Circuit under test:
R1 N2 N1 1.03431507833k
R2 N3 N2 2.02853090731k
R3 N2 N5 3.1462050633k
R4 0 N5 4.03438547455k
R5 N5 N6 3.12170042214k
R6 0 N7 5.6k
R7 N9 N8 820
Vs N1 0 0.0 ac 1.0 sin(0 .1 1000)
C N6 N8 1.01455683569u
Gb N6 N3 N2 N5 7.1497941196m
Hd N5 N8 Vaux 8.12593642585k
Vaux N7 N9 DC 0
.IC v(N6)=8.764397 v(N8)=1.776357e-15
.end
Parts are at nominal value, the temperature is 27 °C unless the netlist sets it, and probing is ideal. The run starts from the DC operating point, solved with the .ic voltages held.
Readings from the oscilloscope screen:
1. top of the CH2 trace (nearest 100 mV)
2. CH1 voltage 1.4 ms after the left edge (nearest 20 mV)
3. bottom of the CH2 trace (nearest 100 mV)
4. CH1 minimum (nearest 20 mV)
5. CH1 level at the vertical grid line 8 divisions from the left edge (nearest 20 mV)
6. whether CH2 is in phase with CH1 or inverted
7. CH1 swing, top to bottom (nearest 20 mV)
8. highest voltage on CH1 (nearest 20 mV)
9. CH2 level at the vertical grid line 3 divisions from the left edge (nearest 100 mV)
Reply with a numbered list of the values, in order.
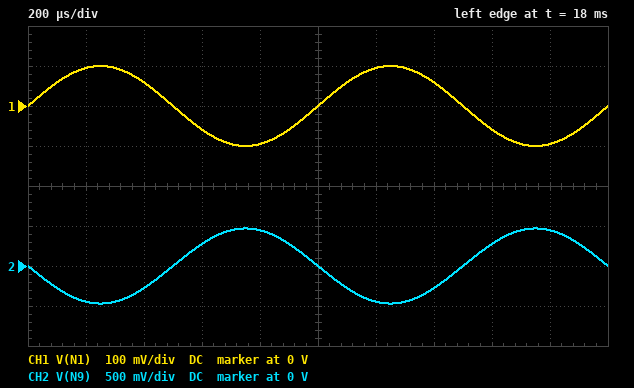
1. 500 mV
2. 60 mV
3. -500 mV
4. -100 mV
5. -60 mV
6. inverted
7. 200 mV
8. 100 mV
9. 300 mV
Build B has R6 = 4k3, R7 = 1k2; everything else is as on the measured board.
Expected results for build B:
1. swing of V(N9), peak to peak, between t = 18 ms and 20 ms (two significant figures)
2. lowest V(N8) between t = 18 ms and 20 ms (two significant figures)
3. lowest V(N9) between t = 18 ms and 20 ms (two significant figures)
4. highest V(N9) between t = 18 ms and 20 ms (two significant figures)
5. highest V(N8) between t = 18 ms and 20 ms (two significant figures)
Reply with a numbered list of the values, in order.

1. 370 mV
2. -240 mV
3. -190 mV
4. 190 mV
5. 240 mV
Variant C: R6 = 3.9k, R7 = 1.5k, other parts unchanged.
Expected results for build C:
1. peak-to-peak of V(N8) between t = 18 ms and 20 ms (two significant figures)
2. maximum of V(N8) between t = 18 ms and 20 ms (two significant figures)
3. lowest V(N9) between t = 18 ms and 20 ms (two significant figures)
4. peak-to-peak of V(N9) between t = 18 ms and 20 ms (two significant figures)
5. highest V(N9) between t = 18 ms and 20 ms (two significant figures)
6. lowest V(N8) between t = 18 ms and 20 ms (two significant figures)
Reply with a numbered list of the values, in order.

1. 440 mV
2. 220 mV
3. -160 mV
4. 320 mV
5. 160 mV
6. -220 mV
